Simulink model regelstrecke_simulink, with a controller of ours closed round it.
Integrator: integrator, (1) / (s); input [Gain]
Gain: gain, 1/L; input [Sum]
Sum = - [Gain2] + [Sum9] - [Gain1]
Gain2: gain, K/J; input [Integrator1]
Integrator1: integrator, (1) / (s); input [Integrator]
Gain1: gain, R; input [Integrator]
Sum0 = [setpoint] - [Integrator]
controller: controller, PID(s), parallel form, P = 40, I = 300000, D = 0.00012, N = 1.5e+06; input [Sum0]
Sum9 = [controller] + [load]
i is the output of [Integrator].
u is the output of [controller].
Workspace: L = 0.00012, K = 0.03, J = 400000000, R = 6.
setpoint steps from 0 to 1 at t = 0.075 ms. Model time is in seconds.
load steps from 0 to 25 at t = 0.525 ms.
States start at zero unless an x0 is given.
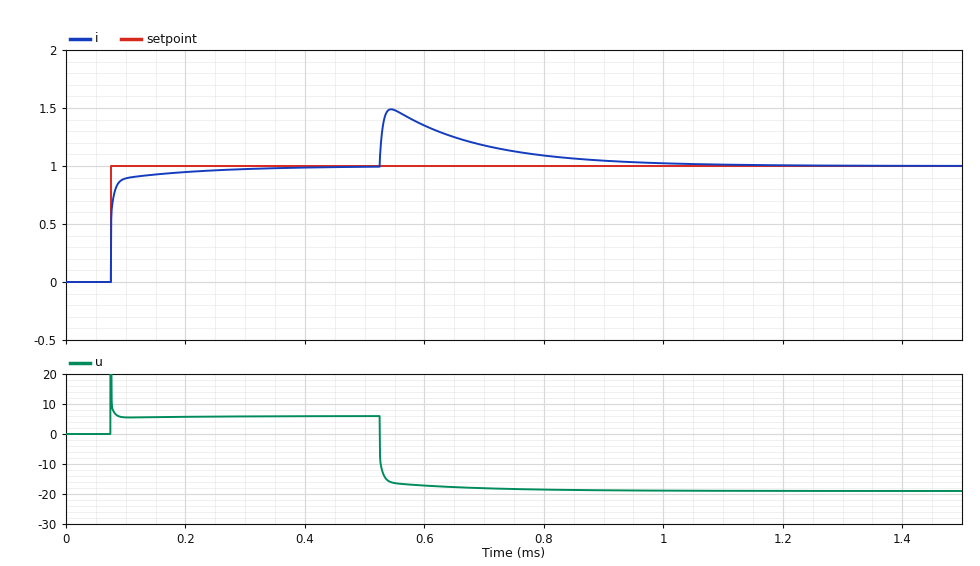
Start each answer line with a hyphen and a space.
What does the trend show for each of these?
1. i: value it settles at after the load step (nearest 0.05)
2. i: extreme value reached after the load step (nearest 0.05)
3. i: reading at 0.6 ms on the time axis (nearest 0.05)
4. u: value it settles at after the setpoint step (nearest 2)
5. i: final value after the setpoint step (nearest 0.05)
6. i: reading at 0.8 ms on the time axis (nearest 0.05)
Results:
- 1.00
- 1.50
- 1.35
- 6
- 1.00
- 1.10
